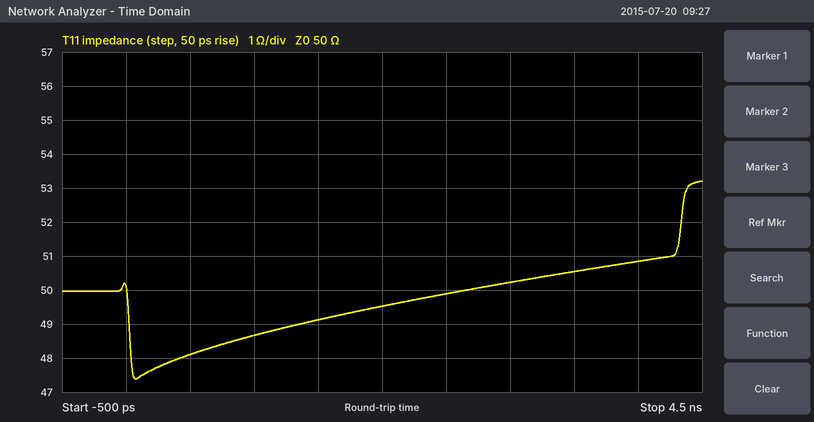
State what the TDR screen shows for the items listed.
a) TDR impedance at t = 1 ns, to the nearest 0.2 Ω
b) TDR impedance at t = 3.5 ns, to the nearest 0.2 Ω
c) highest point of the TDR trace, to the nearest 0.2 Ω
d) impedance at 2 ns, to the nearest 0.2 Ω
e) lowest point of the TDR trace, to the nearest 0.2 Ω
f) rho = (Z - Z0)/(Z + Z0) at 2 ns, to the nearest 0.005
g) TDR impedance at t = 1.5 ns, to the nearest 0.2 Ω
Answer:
48.6 Ω
50.6 Ω
53.2 Ω
49.6 Ω
47.4 Ω
-0.005
49.2 Ω
